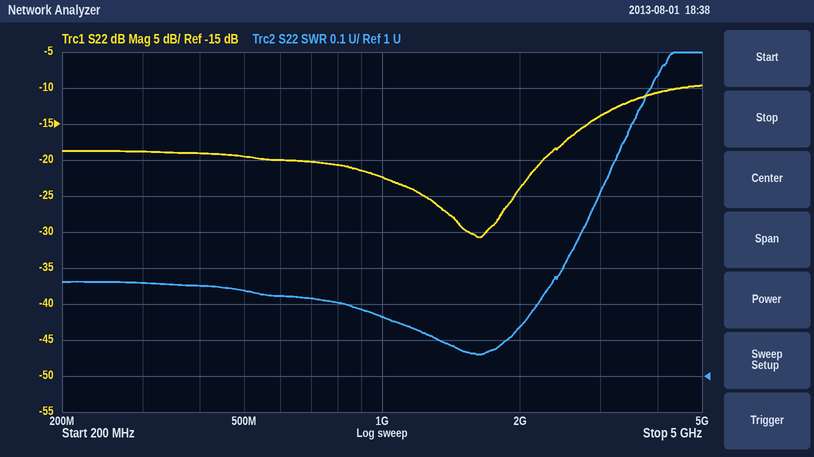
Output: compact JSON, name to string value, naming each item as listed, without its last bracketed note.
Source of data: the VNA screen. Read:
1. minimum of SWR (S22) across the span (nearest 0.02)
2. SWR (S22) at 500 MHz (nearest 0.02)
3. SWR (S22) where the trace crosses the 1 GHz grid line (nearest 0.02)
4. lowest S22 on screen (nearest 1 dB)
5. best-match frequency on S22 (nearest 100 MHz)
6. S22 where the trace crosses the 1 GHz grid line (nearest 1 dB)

{"minimum of SWR (S22) across the span": "1.06", "SWR (S22) at 500 MHz": "1.24", "SWR (S22) where the trace crosses the 1 GHz grid line": "1.16", "lowest S22 on screen": "-31 dB", "best-match frequency on S22": "1.6 GHz", "S22 where the trace crosses the 1 GHz grid line": "-22 dB"}
